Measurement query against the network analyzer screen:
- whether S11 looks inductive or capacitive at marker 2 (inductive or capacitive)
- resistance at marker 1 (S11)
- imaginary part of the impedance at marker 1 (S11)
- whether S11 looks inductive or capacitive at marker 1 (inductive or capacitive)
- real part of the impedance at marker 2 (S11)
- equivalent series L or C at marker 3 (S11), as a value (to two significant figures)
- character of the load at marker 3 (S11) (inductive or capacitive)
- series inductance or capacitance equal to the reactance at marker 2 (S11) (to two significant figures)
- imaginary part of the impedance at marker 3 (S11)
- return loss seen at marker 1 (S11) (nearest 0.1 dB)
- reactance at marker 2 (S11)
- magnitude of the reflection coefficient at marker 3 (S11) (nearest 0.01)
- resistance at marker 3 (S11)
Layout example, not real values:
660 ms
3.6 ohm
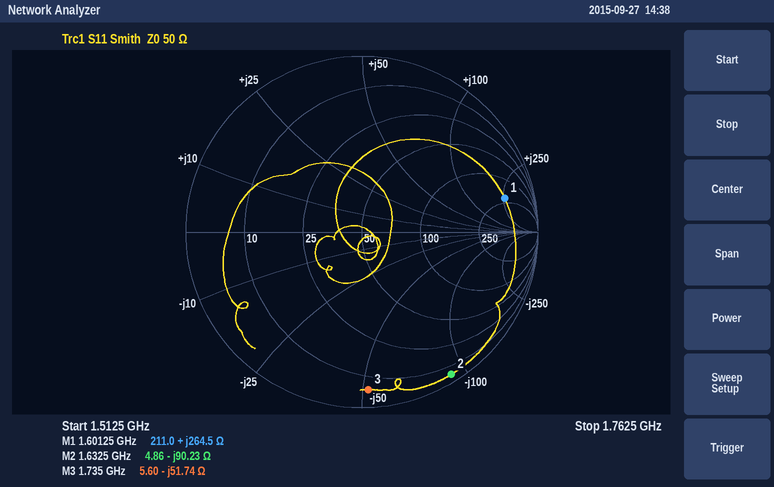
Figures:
capacitive
211.0 Ω
+264.5 Ω
inductive
4.86 Ω
1.8 pF
capacitive
1.1 pF
-51.74 Ω
1.6 dB
-90.23 Ω
0.90
5.60 Ω
